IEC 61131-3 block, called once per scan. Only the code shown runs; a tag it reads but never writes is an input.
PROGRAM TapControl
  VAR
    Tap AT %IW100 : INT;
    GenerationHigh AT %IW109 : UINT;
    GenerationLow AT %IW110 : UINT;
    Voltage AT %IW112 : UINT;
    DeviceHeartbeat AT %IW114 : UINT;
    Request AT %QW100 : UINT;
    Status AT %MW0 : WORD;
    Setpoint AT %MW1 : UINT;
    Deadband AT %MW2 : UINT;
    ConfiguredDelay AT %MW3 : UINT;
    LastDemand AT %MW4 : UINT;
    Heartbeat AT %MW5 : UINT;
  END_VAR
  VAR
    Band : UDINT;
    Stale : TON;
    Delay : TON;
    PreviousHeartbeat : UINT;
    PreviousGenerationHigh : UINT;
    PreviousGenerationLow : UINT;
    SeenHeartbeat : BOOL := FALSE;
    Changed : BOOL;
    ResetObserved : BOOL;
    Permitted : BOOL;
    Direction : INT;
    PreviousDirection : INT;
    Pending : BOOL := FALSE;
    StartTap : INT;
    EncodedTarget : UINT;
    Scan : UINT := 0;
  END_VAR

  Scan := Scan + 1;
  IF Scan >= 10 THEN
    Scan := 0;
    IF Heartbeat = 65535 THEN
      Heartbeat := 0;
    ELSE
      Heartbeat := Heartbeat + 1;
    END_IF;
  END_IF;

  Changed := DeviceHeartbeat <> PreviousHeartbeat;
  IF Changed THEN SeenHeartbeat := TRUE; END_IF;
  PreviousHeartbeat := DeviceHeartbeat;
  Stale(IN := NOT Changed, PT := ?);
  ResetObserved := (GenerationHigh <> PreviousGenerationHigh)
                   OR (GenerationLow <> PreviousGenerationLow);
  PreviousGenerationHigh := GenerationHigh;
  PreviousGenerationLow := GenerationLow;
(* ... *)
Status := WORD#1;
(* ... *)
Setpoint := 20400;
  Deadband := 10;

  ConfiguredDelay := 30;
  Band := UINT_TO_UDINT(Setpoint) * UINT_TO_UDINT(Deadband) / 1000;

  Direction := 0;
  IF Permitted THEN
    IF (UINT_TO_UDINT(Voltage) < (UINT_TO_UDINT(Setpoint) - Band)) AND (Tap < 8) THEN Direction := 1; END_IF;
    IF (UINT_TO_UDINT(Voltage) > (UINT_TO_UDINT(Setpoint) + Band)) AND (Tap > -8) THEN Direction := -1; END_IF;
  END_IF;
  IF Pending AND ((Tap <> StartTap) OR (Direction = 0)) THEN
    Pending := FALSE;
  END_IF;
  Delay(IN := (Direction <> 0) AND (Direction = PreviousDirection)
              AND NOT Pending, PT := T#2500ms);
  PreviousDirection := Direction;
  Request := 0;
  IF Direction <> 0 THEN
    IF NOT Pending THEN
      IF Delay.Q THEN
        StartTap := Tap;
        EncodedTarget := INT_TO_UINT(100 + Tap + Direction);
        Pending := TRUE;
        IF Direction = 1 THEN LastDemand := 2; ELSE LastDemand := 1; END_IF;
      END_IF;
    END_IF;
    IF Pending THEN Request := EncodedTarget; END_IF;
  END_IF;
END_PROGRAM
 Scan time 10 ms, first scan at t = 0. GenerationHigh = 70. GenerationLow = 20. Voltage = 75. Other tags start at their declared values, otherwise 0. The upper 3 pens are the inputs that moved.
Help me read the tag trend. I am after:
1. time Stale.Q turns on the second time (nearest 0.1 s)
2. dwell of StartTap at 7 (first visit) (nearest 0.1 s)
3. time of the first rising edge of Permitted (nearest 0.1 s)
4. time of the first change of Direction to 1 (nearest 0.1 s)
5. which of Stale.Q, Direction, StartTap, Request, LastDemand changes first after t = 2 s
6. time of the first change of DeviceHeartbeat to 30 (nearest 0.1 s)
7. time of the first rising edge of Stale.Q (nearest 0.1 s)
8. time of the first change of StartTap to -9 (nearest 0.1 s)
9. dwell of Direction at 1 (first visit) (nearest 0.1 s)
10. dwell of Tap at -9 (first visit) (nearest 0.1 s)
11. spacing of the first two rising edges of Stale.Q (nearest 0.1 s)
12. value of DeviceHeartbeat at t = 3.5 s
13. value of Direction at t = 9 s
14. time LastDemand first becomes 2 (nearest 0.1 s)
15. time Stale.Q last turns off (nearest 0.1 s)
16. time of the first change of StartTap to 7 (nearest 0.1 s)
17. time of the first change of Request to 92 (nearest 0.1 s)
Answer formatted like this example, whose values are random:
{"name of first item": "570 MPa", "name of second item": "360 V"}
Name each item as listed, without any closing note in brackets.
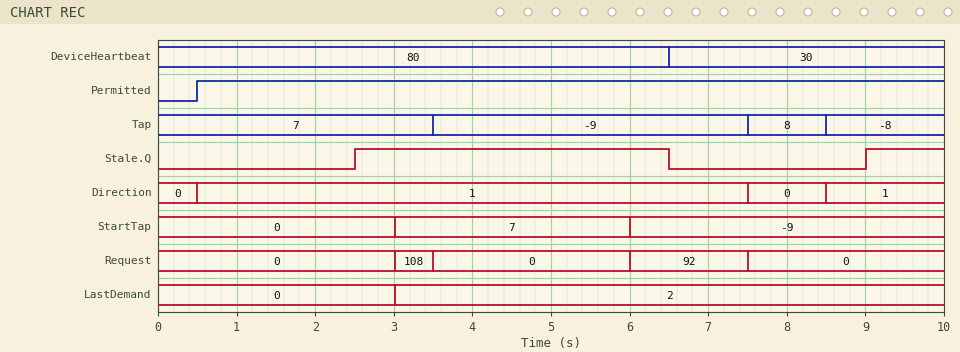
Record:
{"time Stale.Q turns on the second time": "9.0 s", "dwell of StartTap at 7 (first visit)": "3.0 s", "time of the first rising edge of Permitted": "0.5 s", "time of the first change of Direction to 1": "0.5 s", "which of Stale.Q, Direction, StartTap, Request, LastDemand changes first after t = 2 s": "Stale.Q", "time of the first change of DeviceHeartbeat to 30": "6.5 s", "time of the first rising edge of Stale.Q": "2.5 s", "time of the first change of StartTap to -9": "6.0 s", "dwell of Direction at 1 (first visit)": "7.0 s", "dwell of Tap at -9 (first visit)": "4.0 s", "spacing of the first two rising edges of Stale.Q": "6.5 s", "value of DeviceHeartbeat at t = 3.5 s": "80", "value of Direction at t = 9 s": "1", "time LastDemand first becomes 2": "3.0 s", "time Stale.Q last turns off": "6.5 s", "time of the first change of StartTap to 7": "3.0 s", "time of the first change of Request to 92": "6.0 s"}
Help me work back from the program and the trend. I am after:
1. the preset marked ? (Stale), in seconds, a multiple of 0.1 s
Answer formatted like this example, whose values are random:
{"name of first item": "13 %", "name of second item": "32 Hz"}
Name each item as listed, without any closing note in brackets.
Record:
{"the preset marked ? (Stale), in seconds, a multiple of 0.1 s": "2.5 s"}
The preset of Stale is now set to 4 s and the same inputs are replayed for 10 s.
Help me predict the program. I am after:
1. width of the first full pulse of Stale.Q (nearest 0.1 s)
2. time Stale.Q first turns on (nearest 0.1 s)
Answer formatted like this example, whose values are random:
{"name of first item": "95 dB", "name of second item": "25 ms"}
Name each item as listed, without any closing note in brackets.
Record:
{"width of the first full pulse of Stale.Q": "2.5 s", "time Stale.Q first turns on": "4.0 s"}
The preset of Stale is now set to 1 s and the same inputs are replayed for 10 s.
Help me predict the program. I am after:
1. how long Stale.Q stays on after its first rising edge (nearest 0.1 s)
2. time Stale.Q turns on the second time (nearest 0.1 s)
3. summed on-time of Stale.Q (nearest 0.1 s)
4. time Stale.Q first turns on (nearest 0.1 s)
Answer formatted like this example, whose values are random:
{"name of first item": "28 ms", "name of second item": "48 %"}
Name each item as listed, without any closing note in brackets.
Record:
{"how long Stale.Q stays on after its first rising edge": "5.5 s", "time Stale.Q turns on the second time": "7.5 s", "summed on-time of Stale.Q": "8.0 s", "time Stale.Q first turns on": "1.0 s"}
